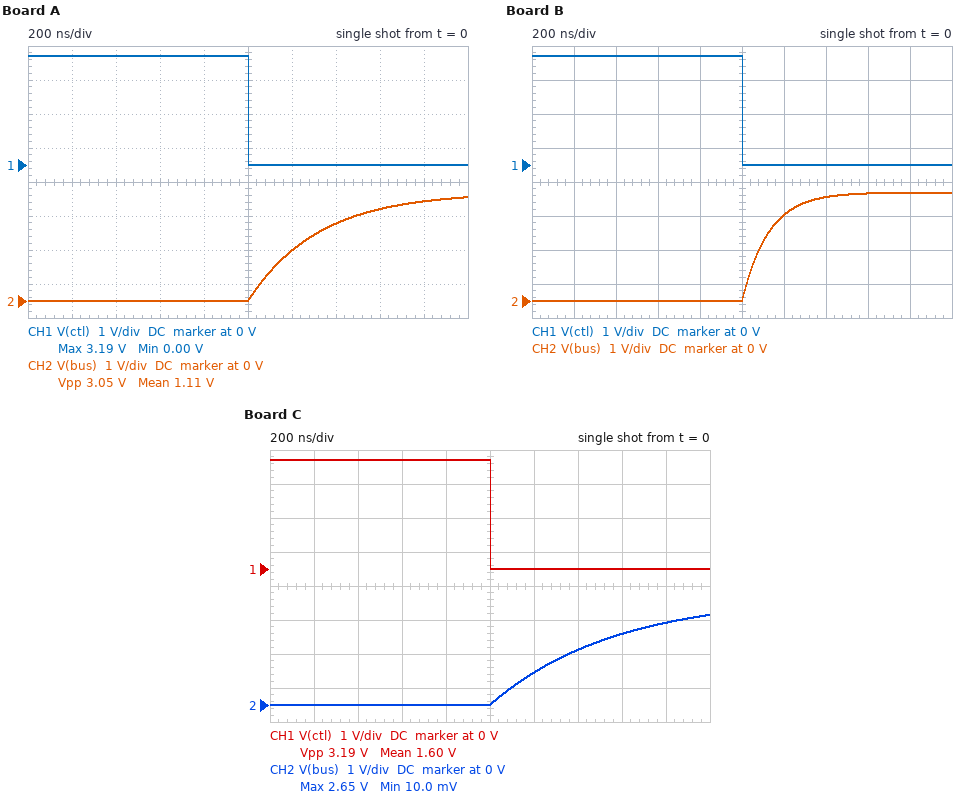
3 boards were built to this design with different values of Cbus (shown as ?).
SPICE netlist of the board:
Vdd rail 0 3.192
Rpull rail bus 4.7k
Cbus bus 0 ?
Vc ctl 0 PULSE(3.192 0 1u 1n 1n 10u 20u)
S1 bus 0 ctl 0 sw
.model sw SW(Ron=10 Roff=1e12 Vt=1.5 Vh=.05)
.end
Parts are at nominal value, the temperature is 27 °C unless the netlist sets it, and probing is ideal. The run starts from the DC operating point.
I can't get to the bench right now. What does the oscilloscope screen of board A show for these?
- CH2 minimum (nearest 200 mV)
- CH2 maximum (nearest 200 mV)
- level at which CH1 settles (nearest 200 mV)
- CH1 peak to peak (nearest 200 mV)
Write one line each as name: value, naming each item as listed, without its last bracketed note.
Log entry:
CH2 minimum: 0 V
CH2 maximum: 3.0 V
level at which CH1 settles: 0 V
CH1 peak to peak: 3.2 V
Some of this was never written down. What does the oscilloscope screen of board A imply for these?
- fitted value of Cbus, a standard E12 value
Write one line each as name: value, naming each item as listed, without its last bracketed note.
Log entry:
fitted value of Cbus, a standard E12 value: 68 pF
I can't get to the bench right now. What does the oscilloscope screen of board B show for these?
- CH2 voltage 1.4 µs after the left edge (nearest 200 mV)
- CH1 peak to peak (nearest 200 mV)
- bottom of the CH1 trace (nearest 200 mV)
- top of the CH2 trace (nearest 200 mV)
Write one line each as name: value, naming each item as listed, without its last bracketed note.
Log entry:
CH2 voltage 1.4 µs after the left edge: 3.0 V
CH1 peak to peak: 3.2 V
bottom of the CH1 trace: 0 V
top of the CH2 trace: 3.2 V
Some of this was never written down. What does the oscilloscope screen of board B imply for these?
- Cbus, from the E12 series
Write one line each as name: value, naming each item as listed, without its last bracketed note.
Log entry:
Cbus, from the E12 series: 27 pF
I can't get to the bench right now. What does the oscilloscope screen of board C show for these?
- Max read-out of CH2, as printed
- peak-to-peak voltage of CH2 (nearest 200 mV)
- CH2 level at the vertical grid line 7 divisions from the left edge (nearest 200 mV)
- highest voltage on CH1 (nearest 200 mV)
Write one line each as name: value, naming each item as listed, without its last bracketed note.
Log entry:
Max read-out of CH2, as printed: 2.65 V
peak-to-peak voltage of CH2: 2.6 V
CH2 level at the vertical grid line 7 divisions from the left edge: 1.6 V
highest voltage on CH1: 3.2 V
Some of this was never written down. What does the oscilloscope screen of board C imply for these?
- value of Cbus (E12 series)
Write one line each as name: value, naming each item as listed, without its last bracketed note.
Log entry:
value of Cbus: 120 pF
